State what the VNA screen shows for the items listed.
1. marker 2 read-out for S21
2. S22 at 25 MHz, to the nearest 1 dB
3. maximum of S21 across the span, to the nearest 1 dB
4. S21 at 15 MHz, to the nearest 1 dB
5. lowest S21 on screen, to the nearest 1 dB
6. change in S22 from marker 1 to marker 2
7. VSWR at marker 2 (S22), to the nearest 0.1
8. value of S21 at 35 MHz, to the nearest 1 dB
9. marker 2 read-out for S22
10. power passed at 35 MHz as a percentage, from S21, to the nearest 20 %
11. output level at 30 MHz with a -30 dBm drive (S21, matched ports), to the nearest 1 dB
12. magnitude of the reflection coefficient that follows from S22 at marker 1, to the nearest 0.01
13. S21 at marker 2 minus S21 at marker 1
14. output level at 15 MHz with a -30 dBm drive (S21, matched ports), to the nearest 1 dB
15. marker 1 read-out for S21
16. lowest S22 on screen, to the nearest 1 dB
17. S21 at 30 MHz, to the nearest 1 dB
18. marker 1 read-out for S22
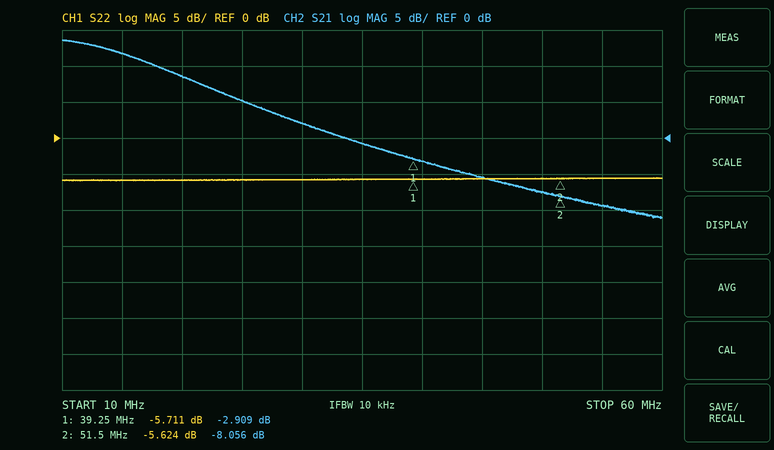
-8.056 dB
-6 dB
14 dB
12 dB
-11 dB
0.087 dB
3.2
-1 dB
-5.624 dB
80 %
-28 dBm
0.52
-5.147 dB
-18 dBm
-2.909 dB
-6 dB
2 dB
-5.711 dB
